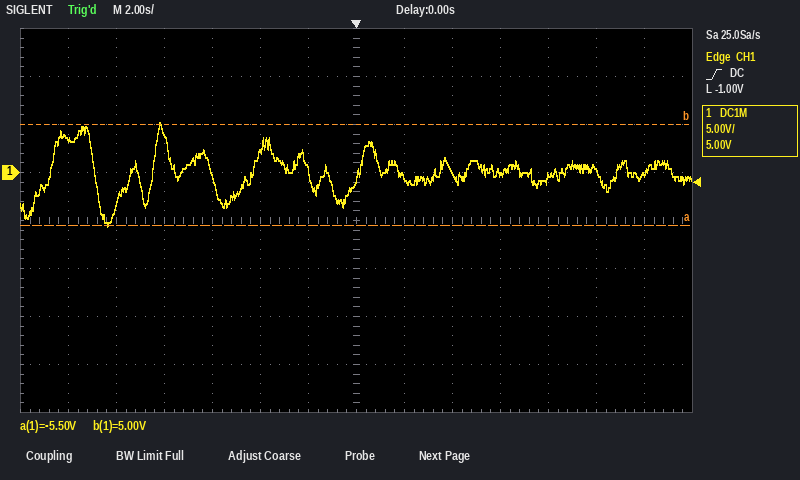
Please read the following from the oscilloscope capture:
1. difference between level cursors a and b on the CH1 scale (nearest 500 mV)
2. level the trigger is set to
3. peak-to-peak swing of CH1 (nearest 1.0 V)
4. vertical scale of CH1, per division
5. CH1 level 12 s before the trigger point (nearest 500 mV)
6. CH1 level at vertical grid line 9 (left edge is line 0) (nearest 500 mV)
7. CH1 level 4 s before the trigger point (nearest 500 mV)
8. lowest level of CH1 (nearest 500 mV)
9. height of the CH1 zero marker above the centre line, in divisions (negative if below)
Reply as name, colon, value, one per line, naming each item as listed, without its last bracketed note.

difference between level cursors a and b on the CH1 scale: 10.5 V
level the trigger is set to: -1.00 V
peak-to-peak swing of CH1: 11.0 V
vertical scale of CH1, per division: 5 V
CH1 level 12 s before the trigger point: 3.5 V
CH1 level at vertical grid line 9 (left edge is line 0): 0.0 V
CH1 level 4 s before the trigger point: 2.0 V
lowest level of CH1: -5.5 V
height of the CH1 zero marker above the centre line, in divisions: +1.0 div
